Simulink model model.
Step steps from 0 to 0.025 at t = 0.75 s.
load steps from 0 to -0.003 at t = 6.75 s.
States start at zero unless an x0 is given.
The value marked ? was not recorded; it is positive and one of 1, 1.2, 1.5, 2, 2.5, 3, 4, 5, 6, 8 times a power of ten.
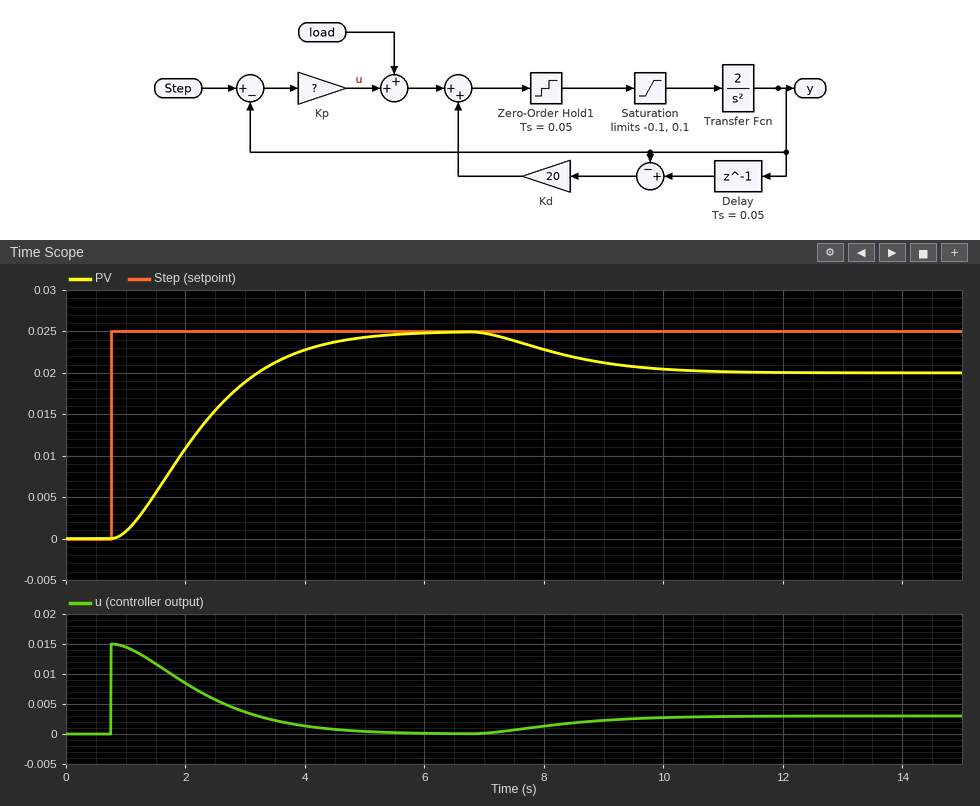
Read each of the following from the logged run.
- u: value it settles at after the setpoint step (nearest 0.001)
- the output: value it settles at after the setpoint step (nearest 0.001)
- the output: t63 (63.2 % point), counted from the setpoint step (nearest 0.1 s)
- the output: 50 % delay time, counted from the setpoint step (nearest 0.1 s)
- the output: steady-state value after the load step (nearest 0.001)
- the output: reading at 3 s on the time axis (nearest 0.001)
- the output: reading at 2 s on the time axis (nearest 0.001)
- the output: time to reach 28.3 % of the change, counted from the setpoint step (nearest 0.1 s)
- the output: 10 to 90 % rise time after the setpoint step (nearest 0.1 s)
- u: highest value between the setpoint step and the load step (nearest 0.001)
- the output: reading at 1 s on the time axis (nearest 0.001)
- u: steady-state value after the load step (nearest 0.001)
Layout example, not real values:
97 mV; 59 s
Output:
0.000; 0.025; 1.8 s; 1.4 s; 0.020; 0.019; 0.011; 0.9 s; 2.7 s; 0.015; 0.001; 0.003
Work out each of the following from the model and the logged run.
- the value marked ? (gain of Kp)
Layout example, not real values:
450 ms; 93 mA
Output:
0.6
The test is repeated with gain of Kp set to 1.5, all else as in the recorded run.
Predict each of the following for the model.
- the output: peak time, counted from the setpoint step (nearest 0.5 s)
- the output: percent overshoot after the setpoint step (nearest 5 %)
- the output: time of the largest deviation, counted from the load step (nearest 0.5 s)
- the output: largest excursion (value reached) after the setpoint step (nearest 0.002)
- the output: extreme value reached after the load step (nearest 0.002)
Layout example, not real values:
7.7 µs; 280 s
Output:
2.0 s; 10 %; 2.0 s; 0.028; 0.022
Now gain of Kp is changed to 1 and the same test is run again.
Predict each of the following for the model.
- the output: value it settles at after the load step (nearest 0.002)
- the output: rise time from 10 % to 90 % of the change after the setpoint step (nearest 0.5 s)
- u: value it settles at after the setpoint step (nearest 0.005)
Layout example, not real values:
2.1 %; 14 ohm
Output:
0.022; 1.5 s; 0.000
